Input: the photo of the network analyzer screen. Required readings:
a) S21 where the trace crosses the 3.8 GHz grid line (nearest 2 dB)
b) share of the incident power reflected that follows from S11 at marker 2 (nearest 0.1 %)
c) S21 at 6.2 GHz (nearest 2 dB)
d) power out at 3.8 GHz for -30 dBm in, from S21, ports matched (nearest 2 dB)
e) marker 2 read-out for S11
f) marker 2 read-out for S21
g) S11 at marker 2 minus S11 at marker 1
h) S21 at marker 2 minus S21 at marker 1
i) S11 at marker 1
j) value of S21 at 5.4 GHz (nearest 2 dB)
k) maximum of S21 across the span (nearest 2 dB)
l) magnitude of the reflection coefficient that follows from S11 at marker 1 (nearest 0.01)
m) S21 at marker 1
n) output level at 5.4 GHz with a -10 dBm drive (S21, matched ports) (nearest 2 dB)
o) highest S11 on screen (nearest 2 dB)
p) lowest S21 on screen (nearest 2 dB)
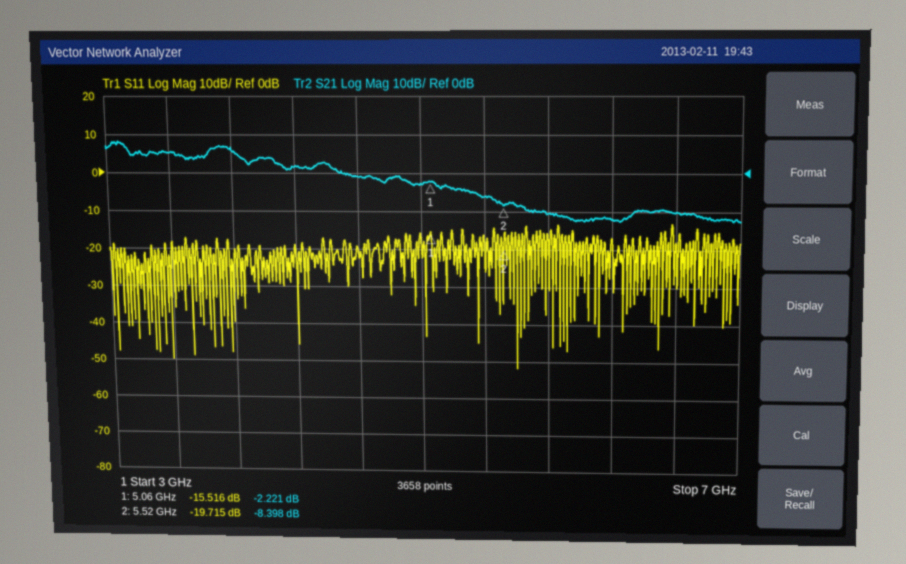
6 dB
1.1 %
-12 dB
-24 dBm
-19.715 dB
-8.398 dB
-4.199 dB
-6.177 dB
-15.516 dB
-6 dB
8 dB
0.17
-2.221 dB
-16 dBm
-14 dB
-12 dB
